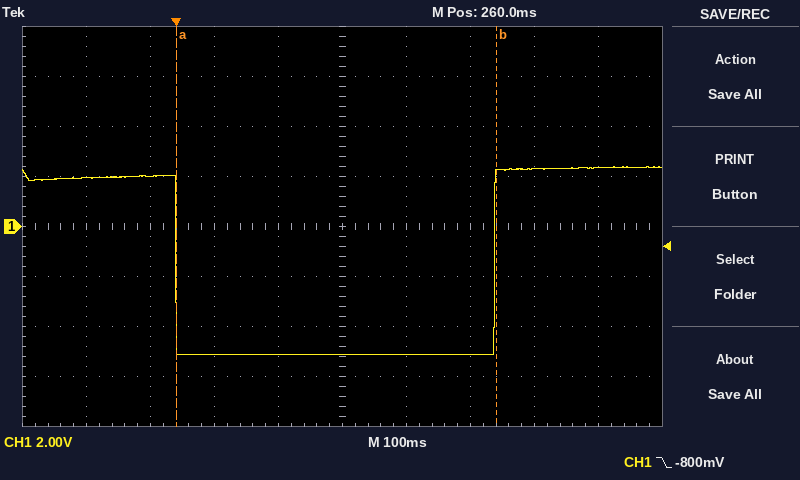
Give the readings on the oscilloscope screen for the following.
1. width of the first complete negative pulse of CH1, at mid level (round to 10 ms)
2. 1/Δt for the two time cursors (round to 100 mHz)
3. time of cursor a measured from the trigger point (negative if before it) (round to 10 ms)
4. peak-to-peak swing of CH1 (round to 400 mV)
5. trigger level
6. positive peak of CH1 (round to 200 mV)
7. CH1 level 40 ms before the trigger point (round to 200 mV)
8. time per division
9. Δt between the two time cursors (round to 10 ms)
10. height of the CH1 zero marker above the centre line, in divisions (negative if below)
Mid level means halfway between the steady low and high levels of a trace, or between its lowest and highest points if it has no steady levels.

500 ms
2.0 Hz
0 ms
7.6 V
-800 mV
2.4 V
2.0 V
100 ms
500 ms
0.0 div
